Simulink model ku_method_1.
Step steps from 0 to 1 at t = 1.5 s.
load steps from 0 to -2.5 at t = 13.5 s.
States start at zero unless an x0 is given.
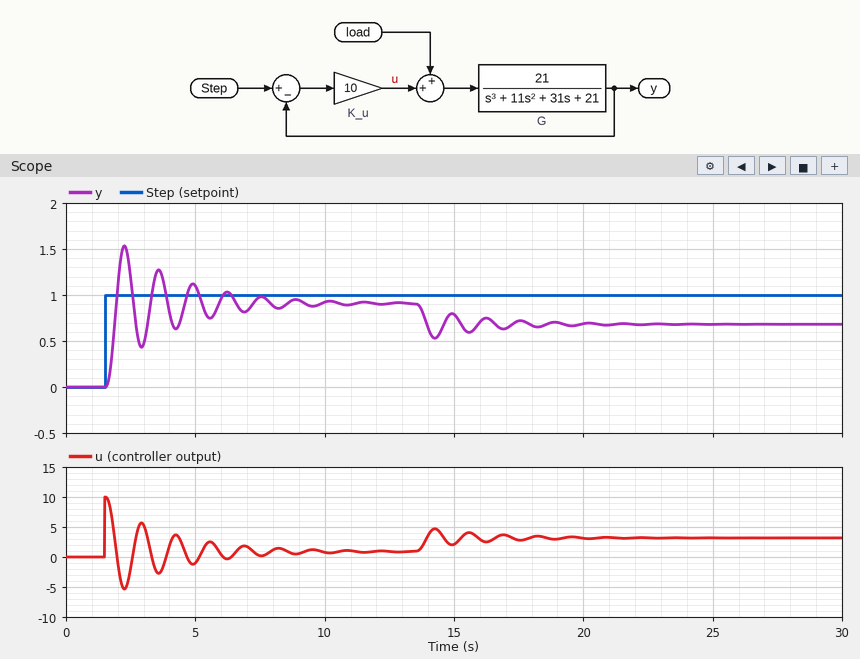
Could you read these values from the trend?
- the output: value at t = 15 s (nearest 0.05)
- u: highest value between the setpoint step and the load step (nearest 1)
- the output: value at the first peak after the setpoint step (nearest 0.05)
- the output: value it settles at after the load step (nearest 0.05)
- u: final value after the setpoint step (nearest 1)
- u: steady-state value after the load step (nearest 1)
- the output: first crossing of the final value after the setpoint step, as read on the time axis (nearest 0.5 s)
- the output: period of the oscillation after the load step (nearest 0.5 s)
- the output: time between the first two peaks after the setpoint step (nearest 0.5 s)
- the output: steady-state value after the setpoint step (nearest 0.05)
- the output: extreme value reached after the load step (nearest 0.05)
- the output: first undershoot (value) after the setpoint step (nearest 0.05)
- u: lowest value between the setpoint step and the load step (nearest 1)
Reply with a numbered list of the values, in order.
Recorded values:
1. 0.80
2. 10
3. 1.55
4. 0.70
5. 1
6. 3
7. 2.0 s
8. 1.5 s
9. 1.5 s
10. 0.90
11. 0.55
12. 0.45
13. -5
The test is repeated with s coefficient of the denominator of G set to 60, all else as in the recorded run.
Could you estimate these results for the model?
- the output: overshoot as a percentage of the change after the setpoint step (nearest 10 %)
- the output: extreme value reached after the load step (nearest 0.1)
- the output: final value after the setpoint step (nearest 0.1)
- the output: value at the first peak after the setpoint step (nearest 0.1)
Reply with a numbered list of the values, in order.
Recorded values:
1. 20 %
2. 0.6
3. 0.9
4. 1.1
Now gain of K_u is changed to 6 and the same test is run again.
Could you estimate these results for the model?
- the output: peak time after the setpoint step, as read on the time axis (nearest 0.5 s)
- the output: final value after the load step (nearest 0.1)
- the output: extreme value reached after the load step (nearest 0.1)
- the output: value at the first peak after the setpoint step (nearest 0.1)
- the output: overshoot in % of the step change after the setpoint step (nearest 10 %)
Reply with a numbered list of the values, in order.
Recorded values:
1. 2.5 s
2. 0.5
3. 0.3
4. 1.3
5. 50 %
